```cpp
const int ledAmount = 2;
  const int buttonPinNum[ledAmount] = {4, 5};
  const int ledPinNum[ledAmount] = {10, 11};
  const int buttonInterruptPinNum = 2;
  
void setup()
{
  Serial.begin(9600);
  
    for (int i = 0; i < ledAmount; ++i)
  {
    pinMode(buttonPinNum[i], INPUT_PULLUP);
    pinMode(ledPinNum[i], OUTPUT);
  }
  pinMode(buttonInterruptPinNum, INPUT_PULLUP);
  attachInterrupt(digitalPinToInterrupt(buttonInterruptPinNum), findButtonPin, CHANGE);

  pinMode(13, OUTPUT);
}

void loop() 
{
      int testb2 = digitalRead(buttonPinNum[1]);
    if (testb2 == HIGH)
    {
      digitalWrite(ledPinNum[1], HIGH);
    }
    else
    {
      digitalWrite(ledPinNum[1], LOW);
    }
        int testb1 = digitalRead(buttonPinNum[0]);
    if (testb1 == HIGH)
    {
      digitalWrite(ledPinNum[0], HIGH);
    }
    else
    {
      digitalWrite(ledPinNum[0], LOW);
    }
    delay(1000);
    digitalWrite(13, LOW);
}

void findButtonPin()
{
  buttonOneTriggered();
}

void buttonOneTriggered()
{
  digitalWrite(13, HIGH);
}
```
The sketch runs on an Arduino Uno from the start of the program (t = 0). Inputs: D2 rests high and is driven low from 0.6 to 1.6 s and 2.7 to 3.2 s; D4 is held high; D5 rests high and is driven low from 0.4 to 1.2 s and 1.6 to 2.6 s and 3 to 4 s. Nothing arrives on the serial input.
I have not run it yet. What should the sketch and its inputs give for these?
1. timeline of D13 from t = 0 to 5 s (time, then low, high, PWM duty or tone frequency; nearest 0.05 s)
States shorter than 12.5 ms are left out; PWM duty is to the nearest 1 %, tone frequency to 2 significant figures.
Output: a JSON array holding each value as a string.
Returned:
["0 s low; 0.6 s high; 1 s low; 1.6 s high; 2 s low; 2.7 s high; 3 s low; 3.2 s high; 4 s low"]
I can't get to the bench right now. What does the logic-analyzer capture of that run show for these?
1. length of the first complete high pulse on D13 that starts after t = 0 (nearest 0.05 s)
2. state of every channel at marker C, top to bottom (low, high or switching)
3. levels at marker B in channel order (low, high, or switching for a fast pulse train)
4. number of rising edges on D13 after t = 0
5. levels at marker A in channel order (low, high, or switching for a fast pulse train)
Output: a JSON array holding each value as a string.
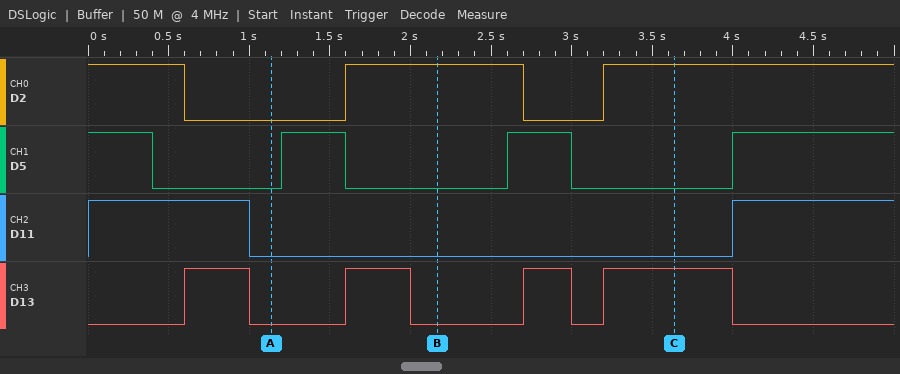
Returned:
["0.40 s", "D2 high, D5 low, D11 low, D13 high", "D2 high, D5 low, D11 low, D13 low", "4", "D2 low, D5 low, D11 low, D13 low"]
